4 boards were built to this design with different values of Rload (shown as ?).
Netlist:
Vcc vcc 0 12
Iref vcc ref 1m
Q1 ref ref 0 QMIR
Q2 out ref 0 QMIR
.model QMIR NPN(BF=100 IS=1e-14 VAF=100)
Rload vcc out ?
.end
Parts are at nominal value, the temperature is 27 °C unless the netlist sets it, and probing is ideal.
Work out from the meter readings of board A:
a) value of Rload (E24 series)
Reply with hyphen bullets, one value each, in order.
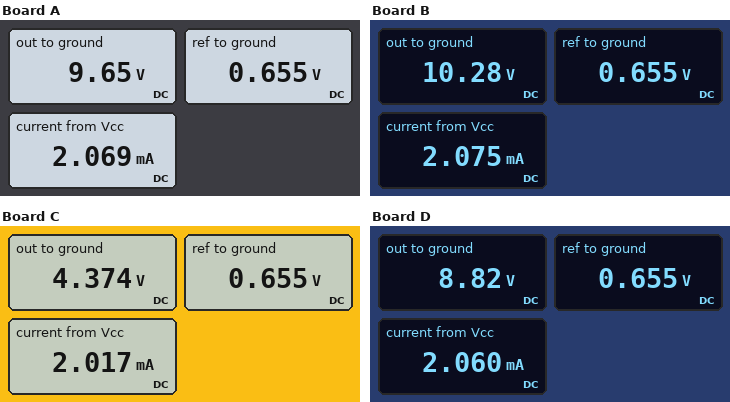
- 2.2 kΩ
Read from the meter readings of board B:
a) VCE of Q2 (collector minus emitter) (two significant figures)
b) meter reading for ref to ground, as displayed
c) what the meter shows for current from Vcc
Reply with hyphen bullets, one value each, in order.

- 10 V
- 0.655 V
- 2.075 mA
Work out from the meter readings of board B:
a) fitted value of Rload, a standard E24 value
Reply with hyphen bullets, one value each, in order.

- 1.6 kΩ
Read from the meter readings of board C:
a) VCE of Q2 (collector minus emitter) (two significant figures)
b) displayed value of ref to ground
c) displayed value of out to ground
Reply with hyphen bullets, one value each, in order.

- 4.4 V
- 0.655 V
- 4.374 V
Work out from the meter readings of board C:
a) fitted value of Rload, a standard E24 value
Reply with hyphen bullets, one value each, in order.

- 7.5 kΩ
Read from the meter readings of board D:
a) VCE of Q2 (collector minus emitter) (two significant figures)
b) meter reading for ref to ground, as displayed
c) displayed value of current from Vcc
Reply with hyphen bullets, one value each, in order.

- 8.8 V
- 0.655 V
- 2.060 mA
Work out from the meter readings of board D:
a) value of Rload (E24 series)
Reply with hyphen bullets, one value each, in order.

- 3 kΩ
